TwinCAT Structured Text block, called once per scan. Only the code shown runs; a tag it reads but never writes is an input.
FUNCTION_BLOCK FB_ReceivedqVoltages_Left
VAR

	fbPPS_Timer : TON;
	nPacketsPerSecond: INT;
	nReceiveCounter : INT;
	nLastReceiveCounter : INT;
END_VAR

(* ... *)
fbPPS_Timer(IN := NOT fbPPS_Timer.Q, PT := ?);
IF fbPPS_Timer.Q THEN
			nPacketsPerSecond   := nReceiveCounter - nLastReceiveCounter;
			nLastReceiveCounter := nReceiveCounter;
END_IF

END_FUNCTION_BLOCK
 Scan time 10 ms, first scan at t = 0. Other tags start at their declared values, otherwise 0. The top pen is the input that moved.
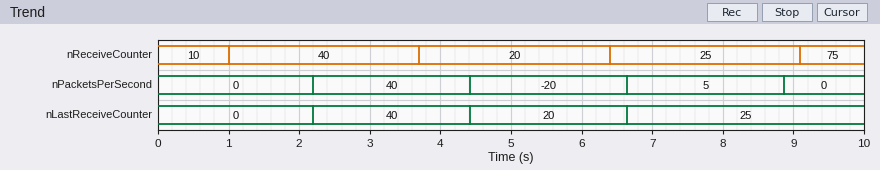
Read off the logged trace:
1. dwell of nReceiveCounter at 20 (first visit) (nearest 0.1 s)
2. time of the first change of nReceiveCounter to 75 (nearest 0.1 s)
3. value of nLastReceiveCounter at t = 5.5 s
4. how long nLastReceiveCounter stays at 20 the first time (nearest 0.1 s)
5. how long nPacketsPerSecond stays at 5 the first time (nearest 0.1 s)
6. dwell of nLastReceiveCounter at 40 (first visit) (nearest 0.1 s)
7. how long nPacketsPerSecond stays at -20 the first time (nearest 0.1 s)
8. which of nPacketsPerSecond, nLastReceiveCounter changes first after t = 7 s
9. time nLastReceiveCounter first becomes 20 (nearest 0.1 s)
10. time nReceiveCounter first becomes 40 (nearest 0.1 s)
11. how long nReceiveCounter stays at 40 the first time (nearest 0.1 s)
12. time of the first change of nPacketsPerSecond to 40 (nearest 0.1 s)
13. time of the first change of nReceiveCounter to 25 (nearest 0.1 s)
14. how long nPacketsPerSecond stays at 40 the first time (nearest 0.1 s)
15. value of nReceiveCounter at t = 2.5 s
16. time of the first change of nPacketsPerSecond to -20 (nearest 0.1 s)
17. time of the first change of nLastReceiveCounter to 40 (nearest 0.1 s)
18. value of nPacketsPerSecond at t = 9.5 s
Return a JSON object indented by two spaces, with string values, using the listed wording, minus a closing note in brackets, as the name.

{
  "dwell of nReceiveCounter at 20 (first visit)": "2.7 s",
  "time of the first change of nReceiveCounter to 75": "9.1 s",
  "value of nLastReceiveCounter at t = 5.5 s": "20",
  "how long nLastReceiveCounter stays at 20 the first time": "2.2 s",
  "how long nPacketsPerSecond stays at 5 the first time": "2.2 s",
  "dwell of nLastReceiveCounter at 40 (first visit)": "2.2 s",
  "how long nPacketsPerSecond stays at -20 the first time": "2.2 s",
  "which of nPacketsPerSecond, nLastReceiveCounter changes first after t = 7 s": "nPacketsPerSecond",
  "time nLastReceiveCounter first becomes 20": "4.4 s",
  "time nReceiveCounter first becomes 40": "1.0 s",
  "how long nReceiveCounter stays at 40 the first time": "2.7 s",
  "time of the first change of nPacketsPerSecond to 40": "2.2 s",
  "time of the first change of nReceiveCounter to 25": "6.4 s",
  "how long nPacketsPerSecond stays at 40 the first time": "2.2 s",
  "value of nReceiveCounter at t = 2.5 s": "40",
  "time of the first change of nPacketsPerSecond to -20": "4.4 s",
  "time of the first change of nLastReceiveCounter to 40": "2.2 s",
  "value of nPacketsPerSecond at t = 9.5 s": "0"
}
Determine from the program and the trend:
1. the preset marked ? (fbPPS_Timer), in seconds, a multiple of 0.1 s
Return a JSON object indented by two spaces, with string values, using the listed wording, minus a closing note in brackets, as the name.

{
  "the preset marked ? (fbPPS_Timer), in seconds, a multiple of 0.1 s": "2.2 s"
}
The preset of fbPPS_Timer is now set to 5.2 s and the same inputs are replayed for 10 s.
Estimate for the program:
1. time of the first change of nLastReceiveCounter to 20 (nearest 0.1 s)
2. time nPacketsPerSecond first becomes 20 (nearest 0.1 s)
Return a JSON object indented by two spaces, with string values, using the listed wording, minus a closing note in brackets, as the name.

{
  "time of the first change of nLastReceiveCounter to 20": "5.2 s",
  "time nPacketsPerSecond first becomes 20": "5.2 s"
}
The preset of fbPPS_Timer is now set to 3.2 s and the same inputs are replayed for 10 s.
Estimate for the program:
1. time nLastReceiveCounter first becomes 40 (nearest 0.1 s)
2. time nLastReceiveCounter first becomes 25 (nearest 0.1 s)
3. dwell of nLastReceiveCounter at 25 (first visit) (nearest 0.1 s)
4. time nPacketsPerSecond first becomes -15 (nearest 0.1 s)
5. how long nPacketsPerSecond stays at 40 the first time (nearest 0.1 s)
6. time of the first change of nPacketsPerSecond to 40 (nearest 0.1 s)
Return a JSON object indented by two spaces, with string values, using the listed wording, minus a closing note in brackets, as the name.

{
  "time nLastReceiveCounter first becomes 40": "3.2 s",
  "time nLastReceiveCounter first becomes 25": "6.4 s",
  "dwell of nLastReceiveCounter at 25 (first visit)": "3.2 s",
  "time nPacketsPerSecond first becomes -15": "6.4 s",
  "how long nPacketsPerSecond stays at 40 the first time": "3.2 s",
  "time of the first change of nPacketsPerSecond to 40": "3.2 s"
}
